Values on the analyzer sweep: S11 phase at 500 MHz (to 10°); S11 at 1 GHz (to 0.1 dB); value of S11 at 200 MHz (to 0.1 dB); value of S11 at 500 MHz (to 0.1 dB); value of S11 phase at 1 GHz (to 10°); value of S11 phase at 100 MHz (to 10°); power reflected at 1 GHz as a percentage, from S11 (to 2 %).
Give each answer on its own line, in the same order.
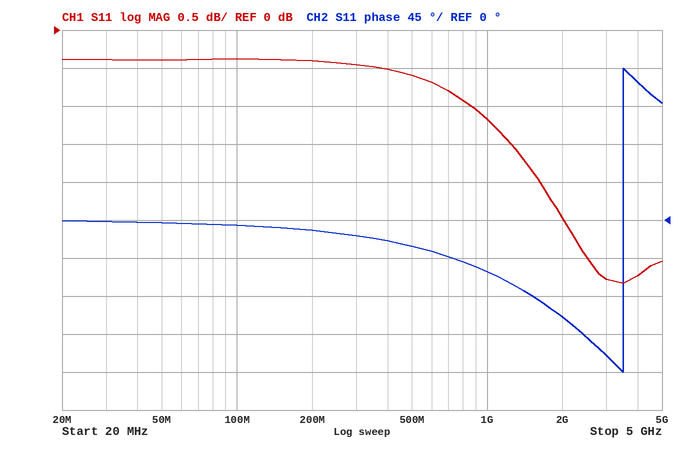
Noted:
-30°
-1.2 dB
-0.4 dB
-0.6 dB
-60°
-10°
76 %
